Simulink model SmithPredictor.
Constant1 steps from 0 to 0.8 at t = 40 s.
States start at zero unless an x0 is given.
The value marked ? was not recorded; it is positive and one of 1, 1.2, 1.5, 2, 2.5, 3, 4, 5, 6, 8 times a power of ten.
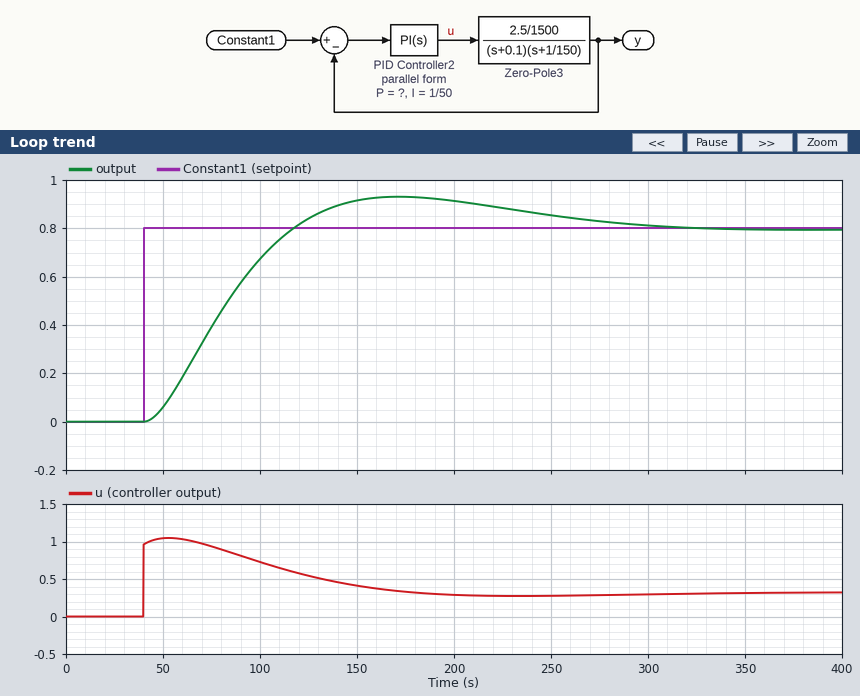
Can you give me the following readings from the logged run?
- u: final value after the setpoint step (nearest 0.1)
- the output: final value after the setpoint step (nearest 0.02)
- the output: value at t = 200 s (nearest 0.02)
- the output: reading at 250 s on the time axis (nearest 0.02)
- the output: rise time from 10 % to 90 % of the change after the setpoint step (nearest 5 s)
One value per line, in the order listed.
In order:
0.3
0.80
0.92
0.86
55 s
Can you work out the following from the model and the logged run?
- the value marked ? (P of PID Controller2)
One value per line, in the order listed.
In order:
1.2
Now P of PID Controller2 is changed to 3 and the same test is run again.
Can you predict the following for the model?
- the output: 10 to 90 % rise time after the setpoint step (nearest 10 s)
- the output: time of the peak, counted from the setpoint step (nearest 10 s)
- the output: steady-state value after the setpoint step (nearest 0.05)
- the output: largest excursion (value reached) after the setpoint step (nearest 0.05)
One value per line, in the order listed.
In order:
30 s
60 s
0.80
0.85
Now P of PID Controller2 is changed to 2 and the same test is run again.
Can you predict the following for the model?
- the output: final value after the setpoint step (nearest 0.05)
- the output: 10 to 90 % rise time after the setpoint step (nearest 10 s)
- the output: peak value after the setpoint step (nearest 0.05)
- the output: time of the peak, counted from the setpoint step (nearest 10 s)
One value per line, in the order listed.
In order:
0.80
40 s
0.85
100 s
